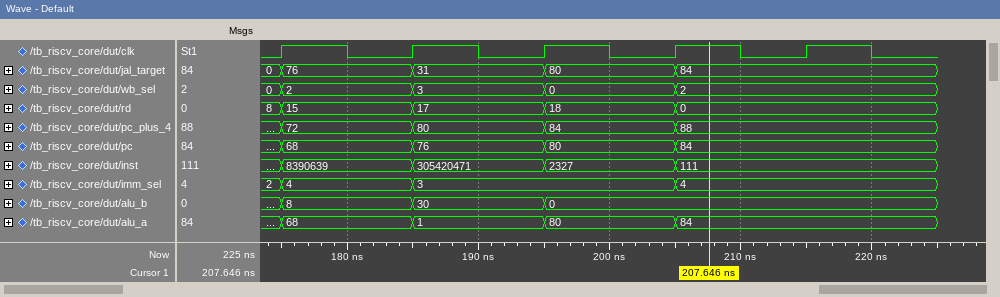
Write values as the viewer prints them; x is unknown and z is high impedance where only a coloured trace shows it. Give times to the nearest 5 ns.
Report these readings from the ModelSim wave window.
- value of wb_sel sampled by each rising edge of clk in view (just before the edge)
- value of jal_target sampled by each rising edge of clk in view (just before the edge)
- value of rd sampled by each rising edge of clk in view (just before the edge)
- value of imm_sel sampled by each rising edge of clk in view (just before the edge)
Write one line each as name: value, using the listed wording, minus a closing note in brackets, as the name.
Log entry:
value of wb_sel sampled by each rising edge of clk in view: 0, 2, 3, 0, 2
value of jal_target sampled by each rising edge of clk in view: 0, 76, 31, 80, 84
value of rd sampled by each rising edge of clk in view: 8, 15, 17, 18, 0
value of imm_sel sampled by each rising edge of clk in view: 2, 4, 3, 3, 4
